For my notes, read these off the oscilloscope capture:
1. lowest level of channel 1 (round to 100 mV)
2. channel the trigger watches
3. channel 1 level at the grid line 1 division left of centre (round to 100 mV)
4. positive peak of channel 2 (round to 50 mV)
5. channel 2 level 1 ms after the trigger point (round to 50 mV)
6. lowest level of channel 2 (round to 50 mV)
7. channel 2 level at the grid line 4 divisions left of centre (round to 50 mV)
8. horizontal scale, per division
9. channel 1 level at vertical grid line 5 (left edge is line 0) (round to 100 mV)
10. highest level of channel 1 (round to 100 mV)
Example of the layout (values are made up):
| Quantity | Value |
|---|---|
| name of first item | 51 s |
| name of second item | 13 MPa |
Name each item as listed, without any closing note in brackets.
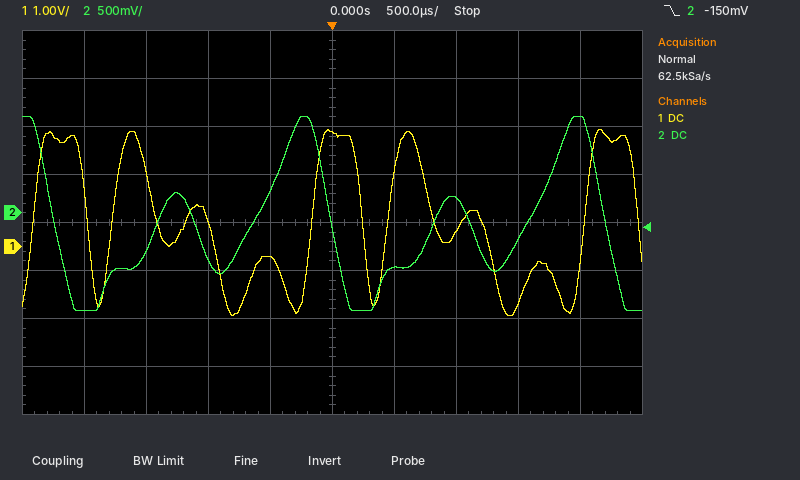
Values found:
| Quantity | Value |
|---|---|
| lowest level of channel 1 | -1.4 V |
| channel the trigger watches | channel 2 |
| channel 1 level at the grid line 1 division left of centre | -200 mV |
| positive peak of channel 2 | 1.00 V |
| channel 2 level 1 ms after the trigger point | 150 mV |
| lowest level of channel 2 | -1.00 V |
| channel 2 level at the grid line 4 divisions left of centre | -1.00 V |
| horizontal scale, per division | 500 µs |
| channel 1 level at vertical grid line 5 (left edge is line 0) | 2.4 V |
| highest level of channel 1 | 2.4 V |
